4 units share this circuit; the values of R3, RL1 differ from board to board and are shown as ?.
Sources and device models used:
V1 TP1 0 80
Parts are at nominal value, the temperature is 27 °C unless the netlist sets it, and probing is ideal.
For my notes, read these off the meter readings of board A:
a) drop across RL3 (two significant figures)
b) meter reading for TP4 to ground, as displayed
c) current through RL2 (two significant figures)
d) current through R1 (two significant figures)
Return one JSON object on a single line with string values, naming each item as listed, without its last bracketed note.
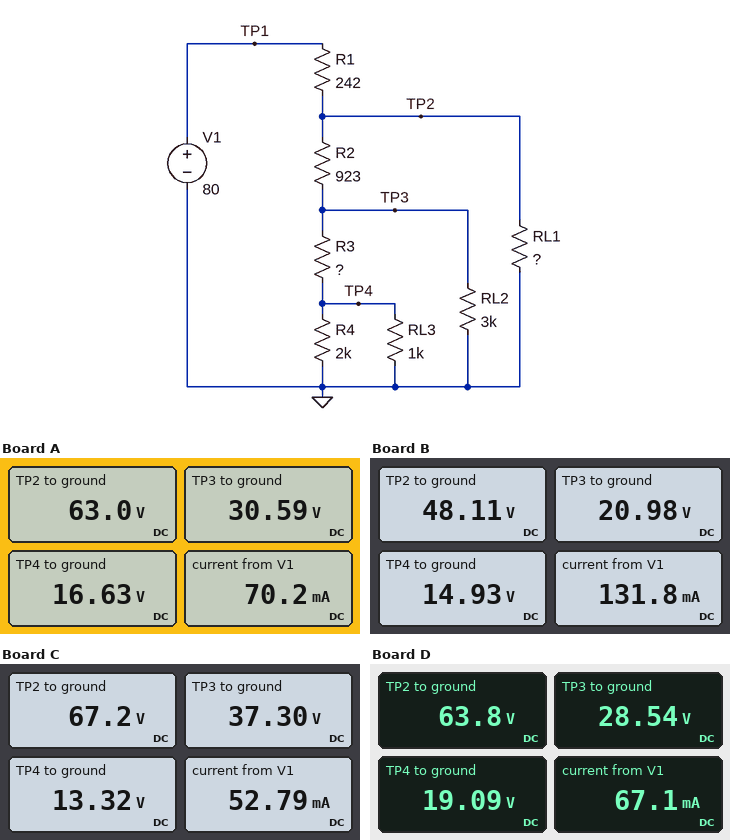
{"drop across RL3": "17 V", "meter reading for TP4 to ground, as displayed": "16.63 V", "current through RL2": "10 mA", "current through R1": "70 mA"}
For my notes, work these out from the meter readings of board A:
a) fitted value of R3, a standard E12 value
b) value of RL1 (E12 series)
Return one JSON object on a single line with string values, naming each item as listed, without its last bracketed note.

{"fitted value of R3, a standard E12 value": "560 Ω", "value of RL1": "1.8 kΩ"}
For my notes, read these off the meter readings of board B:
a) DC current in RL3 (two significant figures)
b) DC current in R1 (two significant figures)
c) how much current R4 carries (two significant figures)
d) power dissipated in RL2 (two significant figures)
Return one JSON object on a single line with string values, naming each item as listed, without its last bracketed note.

{"DC current in RL3": "15 mA", "DC current in R1": "130 mA", "how much current R4 carries": "7.5 mA", "power dissipated in RL2": "150 mW"}
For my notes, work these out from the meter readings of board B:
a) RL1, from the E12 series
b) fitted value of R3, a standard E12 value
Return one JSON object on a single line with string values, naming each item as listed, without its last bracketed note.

{"RL1, from the E12 series": "470 Ω", "fitted value of R3, a standard E12 value": "270 Ω"}
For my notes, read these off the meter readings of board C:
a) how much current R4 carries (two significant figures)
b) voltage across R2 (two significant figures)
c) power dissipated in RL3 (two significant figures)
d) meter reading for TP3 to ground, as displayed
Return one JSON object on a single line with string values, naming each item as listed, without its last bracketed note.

{"how much current R4 carries": "6.7 mA", "voltage across R2": "30 V", "power dissipated in RL3": "180 mW", "meter reading for TP3 to ground, as displayed": "37.30 V"}
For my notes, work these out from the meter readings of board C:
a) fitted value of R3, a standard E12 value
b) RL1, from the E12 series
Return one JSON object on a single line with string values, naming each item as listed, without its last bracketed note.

{"fitted value of R3, a standard E12 value": "1.2 kΩ", "RL1, from the E12 series": "3.3 kΩ"}
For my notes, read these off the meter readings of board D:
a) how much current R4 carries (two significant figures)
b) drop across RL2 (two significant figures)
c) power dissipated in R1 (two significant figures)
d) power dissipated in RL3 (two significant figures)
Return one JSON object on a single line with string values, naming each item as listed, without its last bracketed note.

{"how much current R4 carries": "9.5 mA", "drop across RL2": "29 V", "power dissipated in R1": "1.1 W", "power dissipated in RL3": "360 mW"}
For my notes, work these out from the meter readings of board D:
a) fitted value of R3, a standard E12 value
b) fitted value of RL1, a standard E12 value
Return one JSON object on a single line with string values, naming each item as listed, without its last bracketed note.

{"fitted value of R3, a standard E12 value": "330 Ω", "fitted value of RL1, a standard E12 value": "2.2 kΩ"}
